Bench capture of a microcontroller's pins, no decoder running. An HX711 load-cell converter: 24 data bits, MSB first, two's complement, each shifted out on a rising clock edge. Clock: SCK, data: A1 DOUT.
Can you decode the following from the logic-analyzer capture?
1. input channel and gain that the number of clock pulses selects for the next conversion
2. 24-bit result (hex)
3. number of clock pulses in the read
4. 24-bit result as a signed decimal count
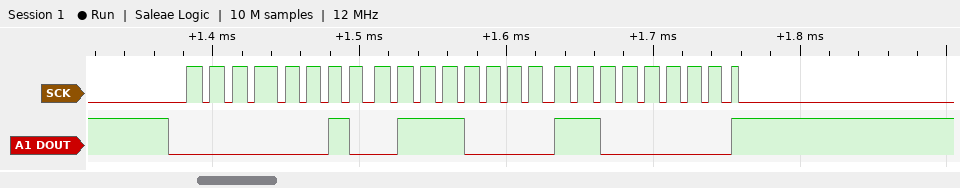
channel A, gain 128
0x0270C0
25
159936
